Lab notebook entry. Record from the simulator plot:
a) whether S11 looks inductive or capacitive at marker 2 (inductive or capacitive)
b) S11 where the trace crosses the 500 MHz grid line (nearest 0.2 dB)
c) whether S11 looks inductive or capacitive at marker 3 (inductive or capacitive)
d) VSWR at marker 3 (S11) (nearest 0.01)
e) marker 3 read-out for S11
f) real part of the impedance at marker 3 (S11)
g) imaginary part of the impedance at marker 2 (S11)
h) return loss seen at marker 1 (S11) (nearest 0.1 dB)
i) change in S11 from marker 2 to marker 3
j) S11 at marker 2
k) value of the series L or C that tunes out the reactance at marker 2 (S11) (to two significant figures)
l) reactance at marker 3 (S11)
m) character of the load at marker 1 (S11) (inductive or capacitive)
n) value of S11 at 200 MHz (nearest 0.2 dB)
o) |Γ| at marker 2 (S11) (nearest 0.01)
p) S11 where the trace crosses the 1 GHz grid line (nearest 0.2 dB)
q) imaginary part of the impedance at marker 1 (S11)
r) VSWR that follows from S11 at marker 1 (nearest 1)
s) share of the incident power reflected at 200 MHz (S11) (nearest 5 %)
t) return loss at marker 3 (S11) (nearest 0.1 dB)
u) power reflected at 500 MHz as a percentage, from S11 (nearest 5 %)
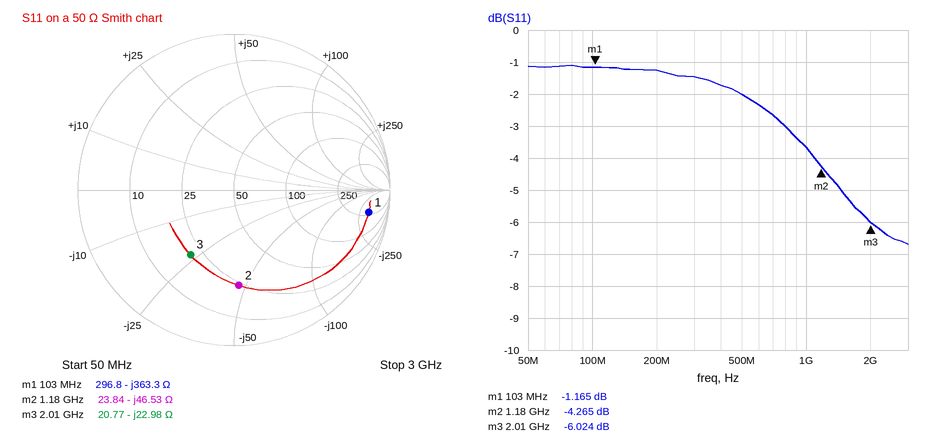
capacitive
-2.0 dB
capacitive
3.00
-6.024 dB
20.77 Ω
-46.53 Ω
1.2 dB
-1.759 dB
-4.265 dB
6.3 nH
-22.98 Ω
capacitive
-1.2 dB
0.61
-3.6 dB
-363.3 Ω
15
75 %
6.0 dB
65 %
